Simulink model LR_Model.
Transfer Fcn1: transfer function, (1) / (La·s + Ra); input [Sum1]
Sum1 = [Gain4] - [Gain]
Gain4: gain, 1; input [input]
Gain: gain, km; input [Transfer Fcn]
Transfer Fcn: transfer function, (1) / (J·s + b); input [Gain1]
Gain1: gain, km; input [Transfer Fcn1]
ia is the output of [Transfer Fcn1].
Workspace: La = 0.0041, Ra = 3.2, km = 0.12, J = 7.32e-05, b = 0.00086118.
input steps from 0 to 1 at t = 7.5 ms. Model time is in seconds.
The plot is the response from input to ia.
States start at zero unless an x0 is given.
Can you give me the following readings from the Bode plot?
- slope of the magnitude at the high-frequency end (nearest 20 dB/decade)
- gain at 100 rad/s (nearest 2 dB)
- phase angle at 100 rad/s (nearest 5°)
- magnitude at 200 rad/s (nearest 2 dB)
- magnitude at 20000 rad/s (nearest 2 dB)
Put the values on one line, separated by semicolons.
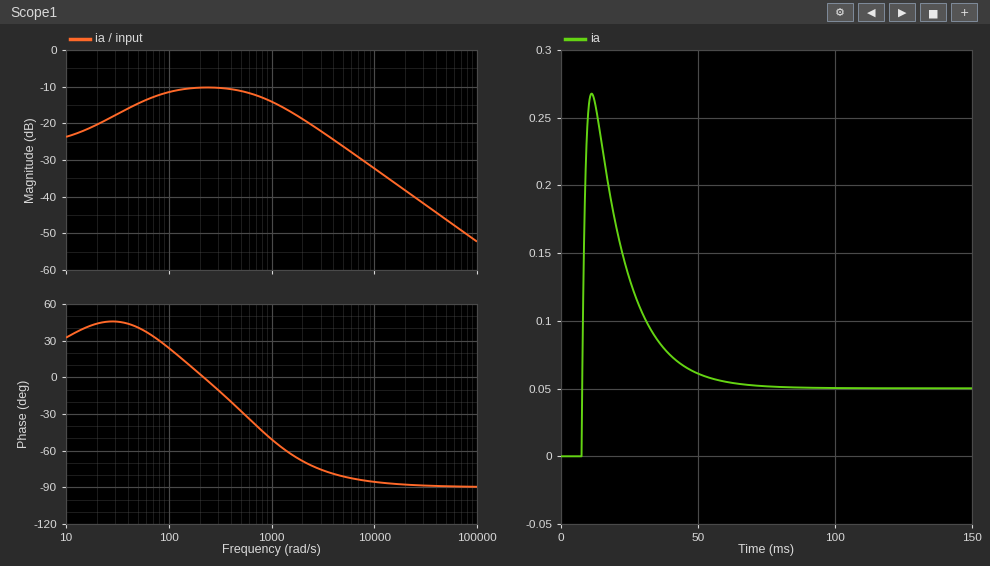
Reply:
-20 dB/decade; -12 dB; 25°; -10 dB; -38 dB
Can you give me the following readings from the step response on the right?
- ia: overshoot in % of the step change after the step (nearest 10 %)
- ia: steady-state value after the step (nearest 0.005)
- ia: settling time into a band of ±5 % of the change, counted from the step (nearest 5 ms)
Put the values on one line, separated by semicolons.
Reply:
430 %; 0.050; 60 ms
